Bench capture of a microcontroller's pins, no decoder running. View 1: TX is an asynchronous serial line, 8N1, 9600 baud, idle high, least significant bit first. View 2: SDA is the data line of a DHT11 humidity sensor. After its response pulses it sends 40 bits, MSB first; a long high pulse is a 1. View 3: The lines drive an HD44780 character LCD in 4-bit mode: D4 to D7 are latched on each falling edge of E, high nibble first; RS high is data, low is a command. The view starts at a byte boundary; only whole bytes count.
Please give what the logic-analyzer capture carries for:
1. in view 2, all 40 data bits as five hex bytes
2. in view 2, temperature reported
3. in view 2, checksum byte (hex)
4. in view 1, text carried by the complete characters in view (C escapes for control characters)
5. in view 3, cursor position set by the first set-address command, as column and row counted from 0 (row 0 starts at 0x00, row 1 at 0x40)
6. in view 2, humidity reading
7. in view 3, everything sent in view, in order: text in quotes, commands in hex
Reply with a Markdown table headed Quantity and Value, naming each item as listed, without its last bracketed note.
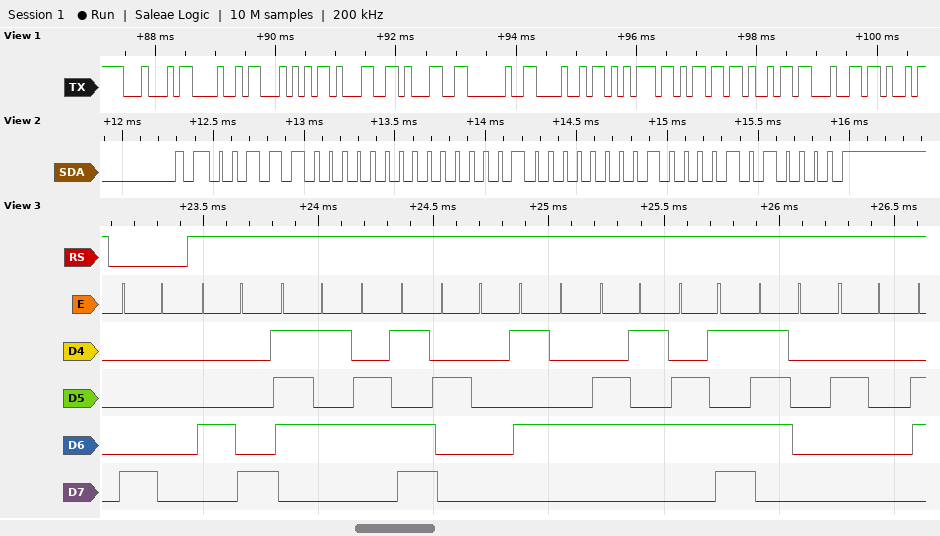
| Quantity | Value |
|---|---|
| in view 2, all 40 data bits as five hex bytes | 38 00 10 08 50 |
| in view 2, temperature reported | 16.8 °C |
| in view 2, checksum byte | 0x50 |
| in view 1, text carried by the complete characters in view | "DHT11 Humid" |
| in view 3, cursor position set by the first set-address command, as column and row counted from 0 | column 0, row 0 |
| in view 2, humidity reading | 56 % |
| in view 3, everything sent in view, in order: text in quotes, commands in hex | 0x80 "Hum Temp " |
